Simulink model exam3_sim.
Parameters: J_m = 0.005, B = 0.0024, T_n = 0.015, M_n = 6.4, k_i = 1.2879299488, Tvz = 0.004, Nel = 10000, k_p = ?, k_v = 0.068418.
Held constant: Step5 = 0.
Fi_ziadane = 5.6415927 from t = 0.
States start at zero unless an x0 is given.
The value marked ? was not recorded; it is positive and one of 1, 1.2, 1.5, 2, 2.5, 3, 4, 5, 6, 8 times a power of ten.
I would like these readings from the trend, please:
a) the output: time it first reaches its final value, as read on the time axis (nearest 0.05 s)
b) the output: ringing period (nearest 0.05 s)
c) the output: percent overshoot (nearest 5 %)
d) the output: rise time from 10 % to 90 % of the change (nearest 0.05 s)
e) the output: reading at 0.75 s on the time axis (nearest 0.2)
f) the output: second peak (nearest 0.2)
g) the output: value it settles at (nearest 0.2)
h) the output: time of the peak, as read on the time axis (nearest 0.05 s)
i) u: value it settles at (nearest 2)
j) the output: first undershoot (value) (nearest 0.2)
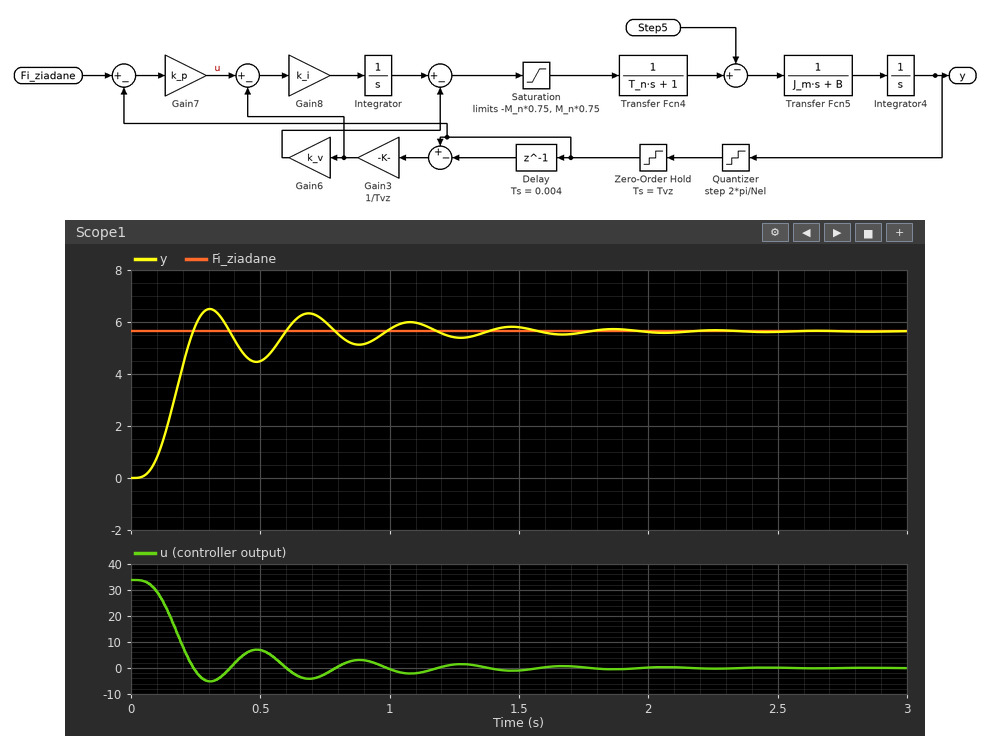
0.25 s
0.40 s
15 %
0.15 s
6.0
6.4
5.6
0.30 s
0
4.4
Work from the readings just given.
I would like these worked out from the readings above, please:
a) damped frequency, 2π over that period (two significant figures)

16 rad/s
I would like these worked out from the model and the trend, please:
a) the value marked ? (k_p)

6
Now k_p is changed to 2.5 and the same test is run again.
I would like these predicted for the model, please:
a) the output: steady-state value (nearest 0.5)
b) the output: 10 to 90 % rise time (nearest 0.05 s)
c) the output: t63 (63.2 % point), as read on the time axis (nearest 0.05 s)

5.5
0.75 s
0.35 s
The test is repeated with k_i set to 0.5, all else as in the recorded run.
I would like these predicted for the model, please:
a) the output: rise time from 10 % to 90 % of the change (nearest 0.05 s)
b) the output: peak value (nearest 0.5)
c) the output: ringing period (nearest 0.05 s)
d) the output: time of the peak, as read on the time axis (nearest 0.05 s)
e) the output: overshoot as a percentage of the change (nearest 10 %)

0.20 s
7.5
0.80 s
0.50 s
30 %
